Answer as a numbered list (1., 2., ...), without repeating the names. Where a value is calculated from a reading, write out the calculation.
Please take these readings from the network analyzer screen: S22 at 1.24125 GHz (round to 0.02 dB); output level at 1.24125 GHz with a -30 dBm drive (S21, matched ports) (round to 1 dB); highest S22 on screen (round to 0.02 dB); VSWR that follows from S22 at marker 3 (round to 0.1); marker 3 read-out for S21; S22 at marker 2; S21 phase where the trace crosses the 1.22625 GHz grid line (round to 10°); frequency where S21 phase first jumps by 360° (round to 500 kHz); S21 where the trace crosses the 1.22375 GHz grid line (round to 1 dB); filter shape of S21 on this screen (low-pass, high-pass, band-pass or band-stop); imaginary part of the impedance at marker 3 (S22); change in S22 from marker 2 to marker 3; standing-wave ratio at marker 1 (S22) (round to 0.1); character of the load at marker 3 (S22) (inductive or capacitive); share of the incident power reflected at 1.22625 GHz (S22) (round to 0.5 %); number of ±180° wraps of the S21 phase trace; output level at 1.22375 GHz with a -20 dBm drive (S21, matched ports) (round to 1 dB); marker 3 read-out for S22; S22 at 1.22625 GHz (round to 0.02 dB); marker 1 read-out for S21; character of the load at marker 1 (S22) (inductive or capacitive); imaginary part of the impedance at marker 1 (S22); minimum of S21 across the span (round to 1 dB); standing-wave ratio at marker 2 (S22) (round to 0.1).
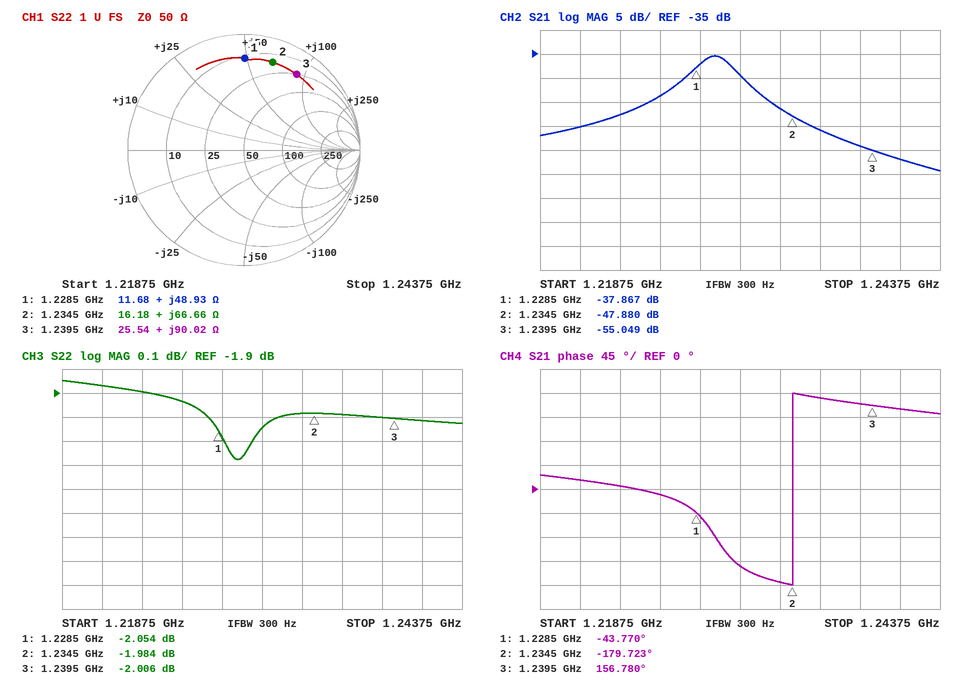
1. -2.02 dB
2. -30 dBm + (-57 dB) = -87 dBm
3. -1.84 dB
4. (1 + 0.7938)/(1 − 0.7938) ≈ 8.7
5. -55.049 dB
6. -1.984 dB
7. -10°
8. 1.2345 GHz
9. -48 dB
10. band-pass
11. +90.02 Ω
12. -2.006 − (-1.984) = -0.022 dB
13. 8.5
14. inductive
15. 10^(-1.94/10) ≈ 64.0 %
16. 1
17. -20 dBm + (-48 dB) = -68 dBm
18. -2.006 dB
19. -1.94 dB
20. -37.867 dB
21. inductive
22. +48.93 Ω
23. -59 dB
24. 8.8
